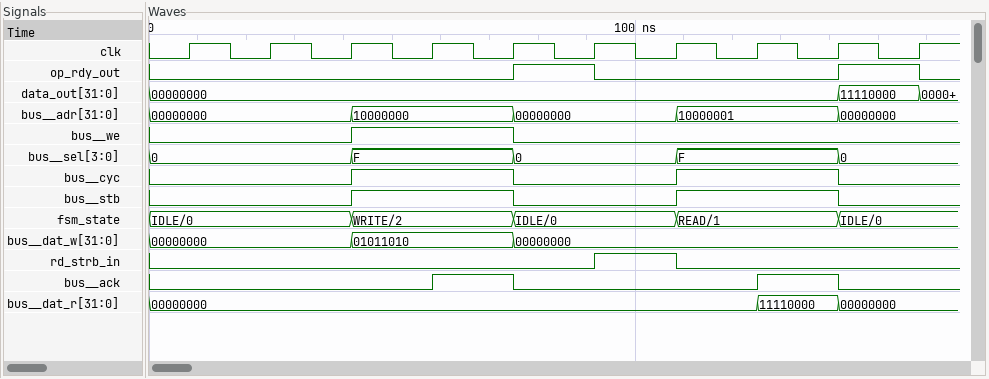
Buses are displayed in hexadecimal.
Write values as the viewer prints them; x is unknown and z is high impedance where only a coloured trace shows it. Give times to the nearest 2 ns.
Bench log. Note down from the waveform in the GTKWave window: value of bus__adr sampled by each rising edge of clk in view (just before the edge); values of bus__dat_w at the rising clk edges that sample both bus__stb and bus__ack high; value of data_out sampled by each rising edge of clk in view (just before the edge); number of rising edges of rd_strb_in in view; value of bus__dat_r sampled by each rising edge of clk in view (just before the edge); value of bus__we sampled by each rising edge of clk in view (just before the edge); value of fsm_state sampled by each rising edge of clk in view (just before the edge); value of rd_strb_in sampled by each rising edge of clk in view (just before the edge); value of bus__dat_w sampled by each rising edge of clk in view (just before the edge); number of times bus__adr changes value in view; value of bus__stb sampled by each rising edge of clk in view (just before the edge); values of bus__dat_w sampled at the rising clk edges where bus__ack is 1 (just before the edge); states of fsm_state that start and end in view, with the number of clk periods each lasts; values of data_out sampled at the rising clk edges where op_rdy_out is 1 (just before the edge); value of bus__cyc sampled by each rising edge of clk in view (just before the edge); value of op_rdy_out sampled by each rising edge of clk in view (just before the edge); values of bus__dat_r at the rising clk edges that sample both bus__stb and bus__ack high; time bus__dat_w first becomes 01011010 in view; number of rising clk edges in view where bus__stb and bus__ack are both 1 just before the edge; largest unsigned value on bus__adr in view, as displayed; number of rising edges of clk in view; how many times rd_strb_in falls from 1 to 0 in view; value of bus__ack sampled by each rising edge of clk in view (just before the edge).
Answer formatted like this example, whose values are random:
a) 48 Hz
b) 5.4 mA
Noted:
a) 00000000, 00000000, 00000000, 10000000, 10000000, 00000000, 00000000, 10000001, 10000001, 00000000
b) 01011010, 00000000
c) 00000000, 00000000, 00000000, 00000000, 00000000, 00000000, 00000000, 00000000, 00000000, 11110000
d) 1
e) 00000000, 00000000, 00000000, 00000000, 00000000, 00000000, 00000000, 00000000, 11110000, 00000000
f) 0 0 0 1 1 0 0 0 0 0
g) IDLE/0, IDLE/0, IDLE/0, WRITE/2, WRITE/2, IDLE/0, IDLE/0, READ/1, READ/1, IDLE/0
h) 0 0 0 0 0 0 1 0 0 0
i) 00000000, 00000000, 00000000, 01011010, 01011010, 00000000, 00000000, 00000000, 00000000, 00000000
j) 4
k) 0 0 0 1 1 0 0 1 1 0
l) 01011010, 00000000
m) WRITE/2: 2, IDLE/0: 2, READ/1: 2
n) 00000000, 11110000
o) 0 0 0 1 1 0 0 1 1 0
p) 0 0 0 0 0 1 0 0 0 1
q) 00000000, 11110000
r) 42 ns
s) 2
t) 10000001
u) 10
v) 1
w) 0 0 0 0 1 0 0 0 1 0
